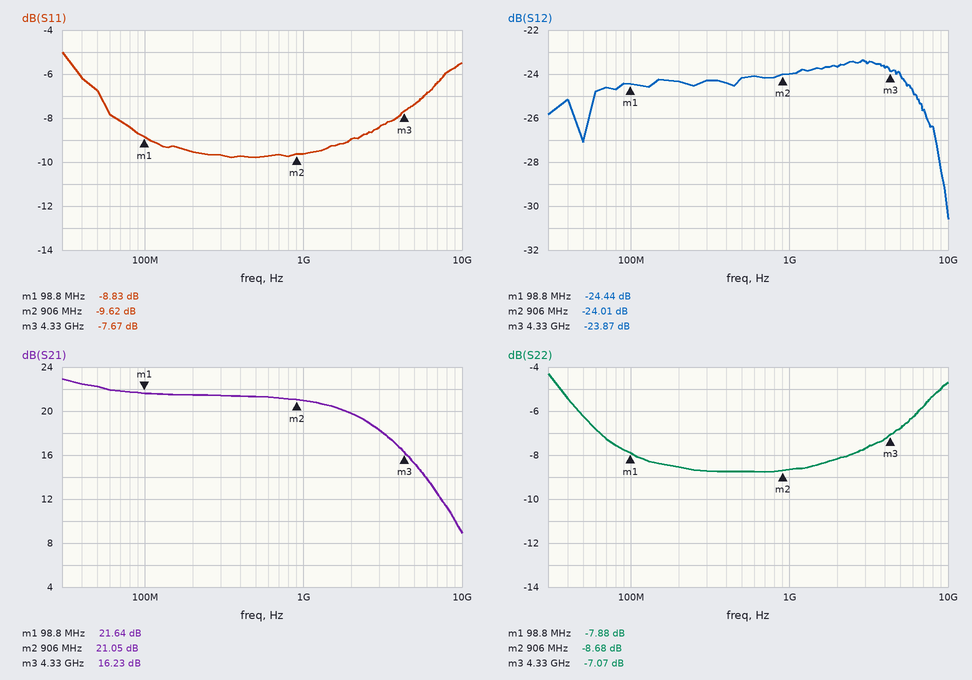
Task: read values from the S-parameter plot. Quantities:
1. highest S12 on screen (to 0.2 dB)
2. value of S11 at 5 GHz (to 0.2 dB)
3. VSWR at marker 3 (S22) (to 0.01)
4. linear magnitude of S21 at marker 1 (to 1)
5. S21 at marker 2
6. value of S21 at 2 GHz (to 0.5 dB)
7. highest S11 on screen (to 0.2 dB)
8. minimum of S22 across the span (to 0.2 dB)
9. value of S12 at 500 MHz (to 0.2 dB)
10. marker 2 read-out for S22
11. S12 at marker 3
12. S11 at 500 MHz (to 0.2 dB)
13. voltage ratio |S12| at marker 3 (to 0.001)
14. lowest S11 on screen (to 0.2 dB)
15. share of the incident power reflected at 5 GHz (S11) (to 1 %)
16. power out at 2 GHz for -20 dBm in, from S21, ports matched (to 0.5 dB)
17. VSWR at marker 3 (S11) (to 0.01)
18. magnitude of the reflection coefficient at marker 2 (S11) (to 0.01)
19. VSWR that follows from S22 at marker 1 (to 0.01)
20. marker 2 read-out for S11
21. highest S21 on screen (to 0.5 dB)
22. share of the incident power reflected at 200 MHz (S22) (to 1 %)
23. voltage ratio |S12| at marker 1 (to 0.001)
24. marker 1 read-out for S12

-23.4 dB
-7.4 dB
2.59
12
21.05 dB
20.0 dB
-5.0 dB
-8.8 dB
-24.2 dB
-8.68 dB
-23.87 dB
-9.8 dB
0.064
-9.8 dB
18 %
0.0 dBm
2.41
0.33
2.35
-9.62 dB
23.0 dB
14 %
0.060
-24.44 dB
